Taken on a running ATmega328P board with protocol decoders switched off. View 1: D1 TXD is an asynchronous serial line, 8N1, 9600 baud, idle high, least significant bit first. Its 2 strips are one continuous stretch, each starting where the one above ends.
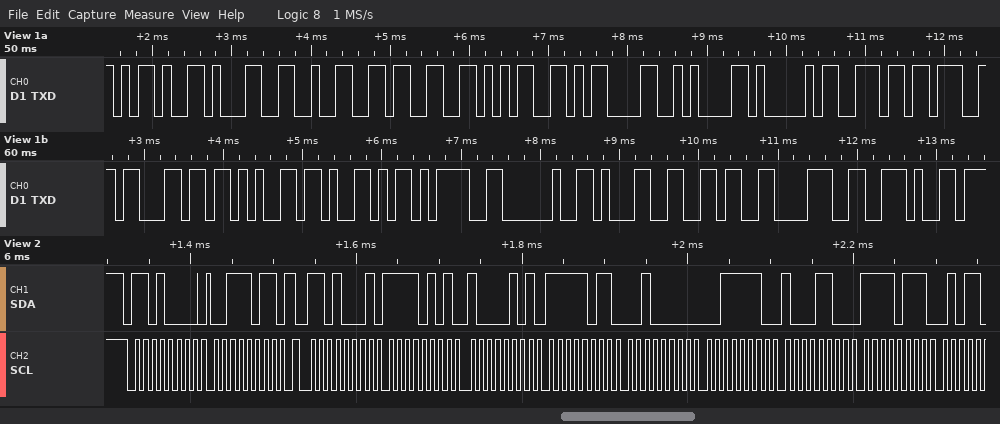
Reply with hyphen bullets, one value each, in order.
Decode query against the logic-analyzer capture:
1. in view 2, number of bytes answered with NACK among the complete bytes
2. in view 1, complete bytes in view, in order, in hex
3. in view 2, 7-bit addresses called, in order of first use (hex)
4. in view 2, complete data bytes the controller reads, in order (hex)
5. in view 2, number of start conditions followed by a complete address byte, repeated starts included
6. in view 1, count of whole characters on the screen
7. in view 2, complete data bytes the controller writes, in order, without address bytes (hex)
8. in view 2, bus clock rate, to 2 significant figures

- 0
- 2D 31 32 33 35 0D 0A 41 6E 67 6C 65 59 3D 20 31 36 38 2E
- 0x68
- F5 85 FB 20 3E 8C F7
- 2
- 19
- 3B
- 100 kHz
